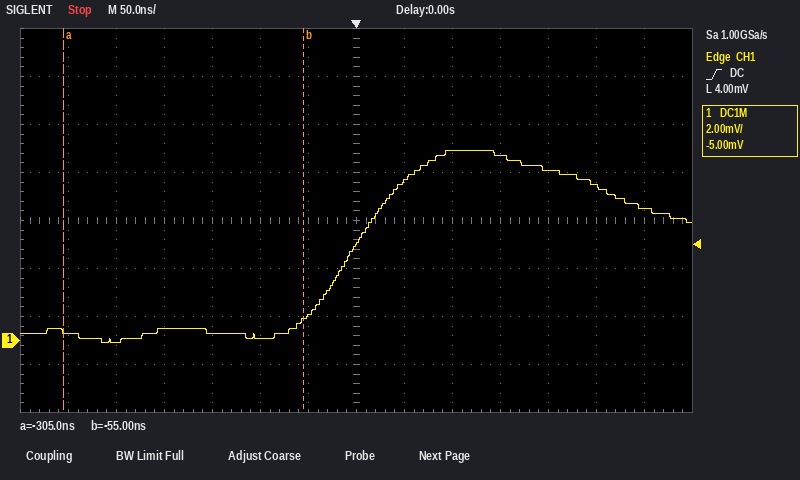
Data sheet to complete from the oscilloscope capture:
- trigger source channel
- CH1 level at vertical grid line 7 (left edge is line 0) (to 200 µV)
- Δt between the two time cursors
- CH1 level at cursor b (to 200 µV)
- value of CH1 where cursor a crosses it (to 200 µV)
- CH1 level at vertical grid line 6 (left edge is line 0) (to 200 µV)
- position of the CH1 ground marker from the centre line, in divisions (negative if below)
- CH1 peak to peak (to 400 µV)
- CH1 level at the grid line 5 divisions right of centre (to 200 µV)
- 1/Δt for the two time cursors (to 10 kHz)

CH1
4.0 mV
250 ns
800 µV
400 µV
1.0 mV
-2.5 div
8.0 mV
6.4 mV
4.00 MHz
